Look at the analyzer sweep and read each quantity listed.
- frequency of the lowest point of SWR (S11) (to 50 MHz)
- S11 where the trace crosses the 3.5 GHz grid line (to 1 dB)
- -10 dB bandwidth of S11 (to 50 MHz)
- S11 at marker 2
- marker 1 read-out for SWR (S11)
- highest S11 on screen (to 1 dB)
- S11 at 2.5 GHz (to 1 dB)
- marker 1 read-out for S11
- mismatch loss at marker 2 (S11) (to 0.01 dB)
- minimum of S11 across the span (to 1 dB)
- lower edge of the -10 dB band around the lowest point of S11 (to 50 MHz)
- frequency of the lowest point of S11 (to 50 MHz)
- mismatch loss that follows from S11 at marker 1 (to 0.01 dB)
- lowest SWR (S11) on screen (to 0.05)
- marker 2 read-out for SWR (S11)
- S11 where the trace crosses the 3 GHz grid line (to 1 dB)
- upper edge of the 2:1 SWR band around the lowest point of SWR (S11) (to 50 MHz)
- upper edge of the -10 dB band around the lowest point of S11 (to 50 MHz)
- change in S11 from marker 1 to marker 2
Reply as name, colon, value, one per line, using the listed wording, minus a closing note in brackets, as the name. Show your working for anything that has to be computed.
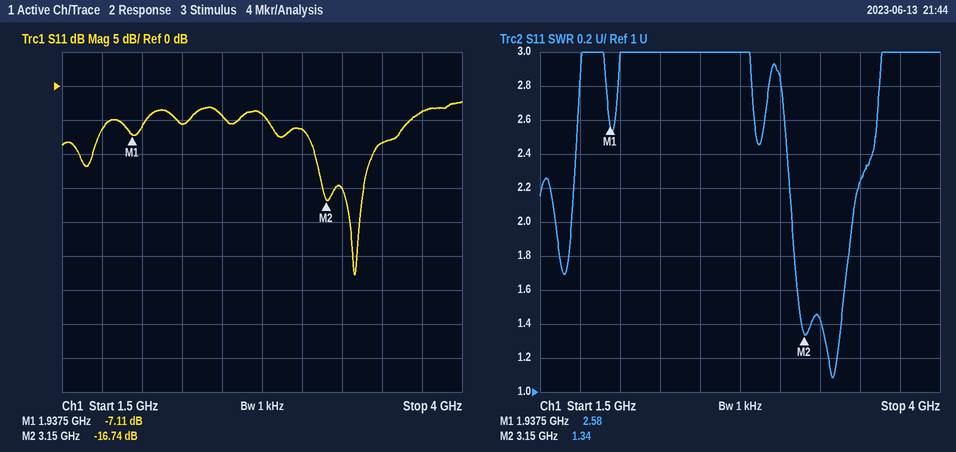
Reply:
frequency of the lowest point of SWR (S11): 3.35 GHz
S11 where the trace crosses the 3.5 GHz grid line: -8 dB
-10 dB bandwidth of S11: 3.45 GHz − 3.10 GHz = 350 MHz
S11 at marker 2: -16.74 dB
marker 1 read-out for SWR: 2.58
highest S11 on screen: -2 dB
S11 at 2.5 GHz: -4 dB
marker 1 read-out for S11: -7.11 dB
mismatch loss at marker 2 (S11): −10 log10(1 − 10^(-16.74/10)) ≈ 0.09 dB
minimum of S11 across the span: -28 dB
lower edge of the -10 dB band around the lowest point of S11: 3.10 GHz
frequency of the lowest point of S11: 3.35 GHz
mismatch loss that follows from S11 at marker 1: −10 log10(1 − 10^(-7.11/10)) ≈ 0.94 dB
lowest SWR (S11) on screen: 1.10
marker 2 read-out for SWR: 1.34
S11 where the trace crosses the 3 GHz grid line: -6 dB
upper edge of the 2:1 SWR band around the lowest point of SWR (S11): 3.45 GHz
upper edge of the -10 dB band around the lowest point of S11: 3.45 GHz
change in S11 from marker 1 to marker 2: -16.74 − (-7.11) = -9.63 dB
